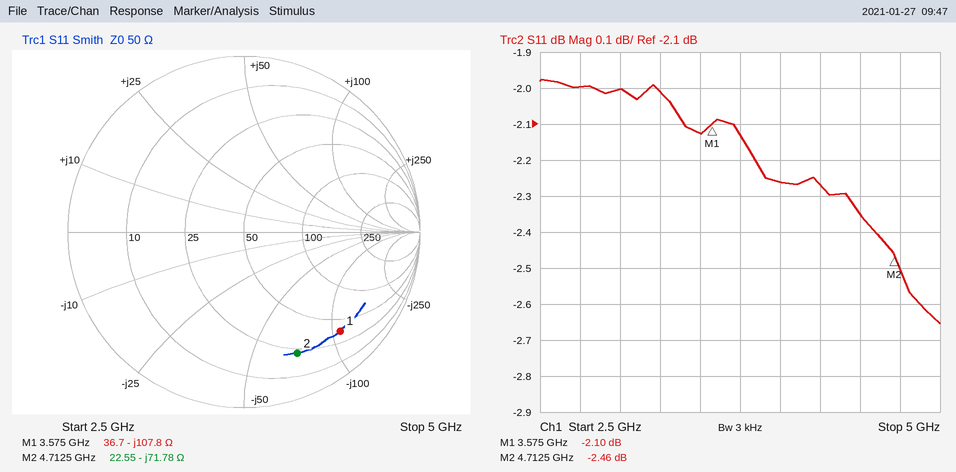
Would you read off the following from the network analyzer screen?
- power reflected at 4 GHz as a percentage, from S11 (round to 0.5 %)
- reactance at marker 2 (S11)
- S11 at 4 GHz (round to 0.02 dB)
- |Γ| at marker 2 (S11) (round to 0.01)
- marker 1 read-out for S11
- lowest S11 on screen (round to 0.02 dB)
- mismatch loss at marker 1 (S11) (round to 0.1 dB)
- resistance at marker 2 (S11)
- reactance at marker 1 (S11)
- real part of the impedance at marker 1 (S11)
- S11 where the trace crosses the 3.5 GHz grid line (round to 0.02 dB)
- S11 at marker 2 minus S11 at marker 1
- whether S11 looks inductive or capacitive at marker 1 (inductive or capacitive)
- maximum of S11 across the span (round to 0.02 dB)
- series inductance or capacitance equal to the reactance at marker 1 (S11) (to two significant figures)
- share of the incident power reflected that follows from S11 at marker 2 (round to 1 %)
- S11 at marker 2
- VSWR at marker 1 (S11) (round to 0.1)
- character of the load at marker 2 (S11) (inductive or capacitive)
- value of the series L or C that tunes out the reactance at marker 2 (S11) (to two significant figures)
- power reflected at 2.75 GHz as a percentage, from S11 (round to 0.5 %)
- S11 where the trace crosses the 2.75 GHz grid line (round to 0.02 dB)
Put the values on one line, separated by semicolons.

59.5 %; -71.78 Ω; -2.26 dB; 0.75; -2.10 dB; -2.66 dB; 4.2 dB; 22.55 Ω; -107.8 Ω; 36.7 Ω; -2.12 dB; -0.36 dB; capacitive; -1.98 dB; 410 fF; 57 %; -2.46 dB; 8.3; capacitive; 2.4 nH; 63.0 %; -2.00 dB
